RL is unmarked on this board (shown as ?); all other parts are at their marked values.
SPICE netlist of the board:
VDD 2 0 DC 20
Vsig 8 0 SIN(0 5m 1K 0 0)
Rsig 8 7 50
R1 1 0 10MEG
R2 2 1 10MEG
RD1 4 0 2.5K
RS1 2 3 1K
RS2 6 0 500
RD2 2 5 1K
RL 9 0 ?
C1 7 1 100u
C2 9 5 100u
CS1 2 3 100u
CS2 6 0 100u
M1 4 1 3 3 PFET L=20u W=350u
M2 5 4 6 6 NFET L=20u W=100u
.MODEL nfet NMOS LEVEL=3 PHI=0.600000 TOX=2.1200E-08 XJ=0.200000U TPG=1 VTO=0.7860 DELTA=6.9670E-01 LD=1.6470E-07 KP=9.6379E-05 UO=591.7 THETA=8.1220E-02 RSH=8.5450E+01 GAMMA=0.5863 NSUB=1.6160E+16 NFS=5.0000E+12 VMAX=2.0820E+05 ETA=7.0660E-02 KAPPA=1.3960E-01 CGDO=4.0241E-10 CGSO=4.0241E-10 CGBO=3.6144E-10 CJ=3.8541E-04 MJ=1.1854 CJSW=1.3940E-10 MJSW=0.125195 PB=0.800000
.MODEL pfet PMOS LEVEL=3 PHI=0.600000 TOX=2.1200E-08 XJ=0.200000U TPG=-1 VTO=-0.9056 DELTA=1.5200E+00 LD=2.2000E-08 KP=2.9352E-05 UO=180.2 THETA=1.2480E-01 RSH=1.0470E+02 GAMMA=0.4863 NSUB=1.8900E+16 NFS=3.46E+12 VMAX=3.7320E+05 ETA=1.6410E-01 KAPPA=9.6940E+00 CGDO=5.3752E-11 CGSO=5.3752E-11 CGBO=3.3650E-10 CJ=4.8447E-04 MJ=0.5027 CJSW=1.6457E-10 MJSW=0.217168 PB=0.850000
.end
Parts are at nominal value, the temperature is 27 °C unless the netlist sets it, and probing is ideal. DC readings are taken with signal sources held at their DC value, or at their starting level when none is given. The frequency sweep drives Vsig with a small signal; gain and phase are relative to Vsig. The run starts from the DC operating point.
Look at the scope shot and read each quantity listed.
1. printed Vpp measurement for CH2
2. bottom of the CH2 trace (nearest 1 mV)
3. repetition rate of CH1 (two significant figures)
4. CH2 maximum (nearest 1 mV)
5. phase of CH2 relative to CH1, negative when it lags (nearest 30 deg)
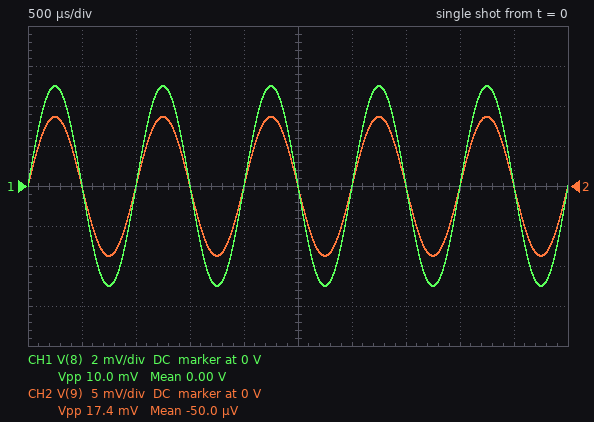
17.4 mV
-9 mV
1.0 kHz
9 mV
0 deg
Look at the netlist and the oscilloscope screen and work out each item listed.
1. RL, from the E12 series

1.5 kΩ
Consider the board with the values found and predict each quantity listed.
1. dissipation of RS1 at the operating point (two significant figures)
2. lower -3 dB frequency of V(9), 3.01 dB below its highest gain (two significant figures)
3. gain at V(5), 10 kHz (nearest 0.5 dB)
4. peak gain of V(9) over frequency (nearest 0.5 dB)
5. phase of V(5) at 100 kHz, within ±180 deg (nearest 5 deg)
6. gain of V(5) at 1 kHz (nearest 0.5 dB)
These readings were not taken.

13 mW
4.6 Hz
5.0 dB
5.0 dB
0 deg
5.0 dB
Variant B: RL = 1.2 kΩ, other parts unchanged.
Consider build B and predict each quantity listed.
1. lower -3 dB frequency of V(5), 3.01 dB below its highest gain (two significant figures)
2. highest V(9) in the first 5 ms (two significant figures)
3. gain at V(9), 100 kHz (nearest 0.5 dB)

4.2 Hz
7.9 mV
4.0 dB
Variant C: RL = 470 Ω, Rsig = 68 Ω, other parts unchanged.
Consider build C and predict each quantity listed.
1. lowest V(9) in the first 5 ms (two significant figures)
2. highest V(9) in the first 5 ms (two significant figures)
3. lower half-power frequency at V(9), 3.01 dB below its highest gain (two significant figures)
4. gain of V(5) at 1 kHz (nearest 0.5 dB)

-4.7 mV
4.6 mV
4.8 Hz
-0.5 dB
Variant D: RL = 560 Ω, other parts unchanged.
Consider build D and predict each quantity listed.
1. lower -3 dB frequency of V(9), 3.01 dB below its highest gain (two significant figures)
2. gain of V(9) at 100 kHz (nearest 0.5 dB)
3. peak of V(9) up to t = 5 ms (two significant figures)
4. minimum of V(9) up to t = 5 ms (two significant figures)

4.7 Hz
0.5 dB
5.2 mV
-5.2 mV
